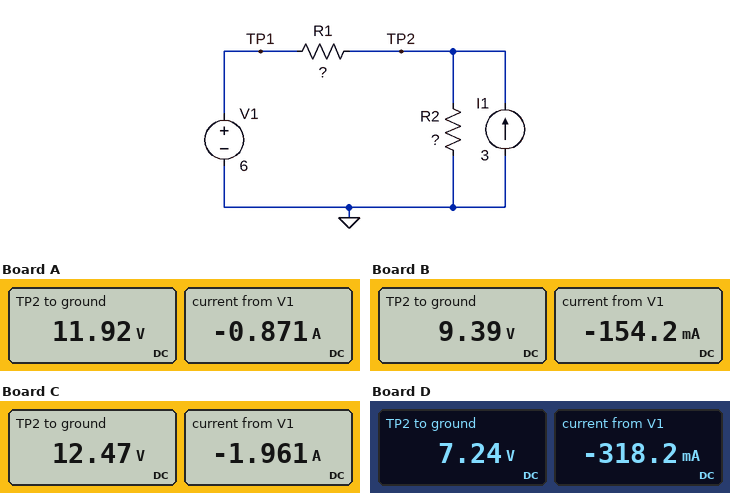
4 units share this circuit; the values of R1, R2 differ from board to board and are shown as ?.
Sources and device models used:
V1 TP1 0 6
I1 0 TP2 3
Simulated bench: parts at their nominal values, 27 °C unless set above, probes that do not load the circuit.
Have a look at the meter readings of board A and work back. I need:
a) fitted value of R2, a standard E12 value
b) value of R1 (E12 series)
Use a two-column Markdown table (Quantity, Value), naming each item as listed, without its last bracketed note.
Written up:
| Quantity | Value |
|---|---|
| fitted value of R2, a standard E12 value | 5.6 Ω |
| value of R1 | 6.8 Ω |
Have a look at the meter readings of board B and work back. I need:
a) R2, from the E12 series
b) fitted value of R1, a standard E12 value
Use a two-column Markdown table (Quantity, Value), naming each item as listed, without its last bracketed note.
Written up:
| Quantity | Value |
|---|---|
| R2, from the E12 series | 3.3 Ω |
| fitted value of R1, a standard E12 value | 22 Ω |
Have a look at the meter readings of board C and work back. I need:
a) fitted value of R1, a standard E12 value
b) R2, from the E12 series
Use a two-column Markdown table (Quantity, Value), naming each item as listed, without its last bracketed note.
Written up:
| Quantity | Value |
|---|---|
| fitted value of R1, a standard E12 value | 3.3 Ω |
| R2, from the E12 series | 12 Ω |
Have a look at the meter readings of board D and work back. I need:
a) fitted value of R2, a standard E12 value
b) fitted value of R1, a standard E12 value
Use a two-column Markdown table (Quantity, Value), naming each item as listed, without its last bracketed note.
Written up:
| Quantity | Value |
|---|---|
| fitted value of R2, a standard E12 value | 2.7 Ω |
| fitted value of R1, a standard E12 value | 3.9 Ω |
